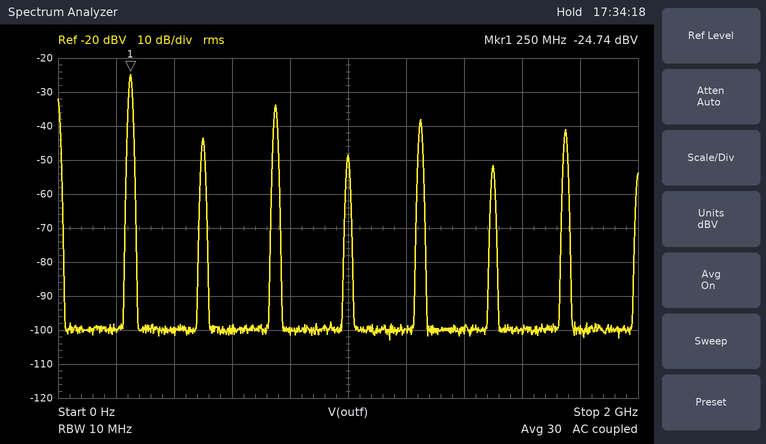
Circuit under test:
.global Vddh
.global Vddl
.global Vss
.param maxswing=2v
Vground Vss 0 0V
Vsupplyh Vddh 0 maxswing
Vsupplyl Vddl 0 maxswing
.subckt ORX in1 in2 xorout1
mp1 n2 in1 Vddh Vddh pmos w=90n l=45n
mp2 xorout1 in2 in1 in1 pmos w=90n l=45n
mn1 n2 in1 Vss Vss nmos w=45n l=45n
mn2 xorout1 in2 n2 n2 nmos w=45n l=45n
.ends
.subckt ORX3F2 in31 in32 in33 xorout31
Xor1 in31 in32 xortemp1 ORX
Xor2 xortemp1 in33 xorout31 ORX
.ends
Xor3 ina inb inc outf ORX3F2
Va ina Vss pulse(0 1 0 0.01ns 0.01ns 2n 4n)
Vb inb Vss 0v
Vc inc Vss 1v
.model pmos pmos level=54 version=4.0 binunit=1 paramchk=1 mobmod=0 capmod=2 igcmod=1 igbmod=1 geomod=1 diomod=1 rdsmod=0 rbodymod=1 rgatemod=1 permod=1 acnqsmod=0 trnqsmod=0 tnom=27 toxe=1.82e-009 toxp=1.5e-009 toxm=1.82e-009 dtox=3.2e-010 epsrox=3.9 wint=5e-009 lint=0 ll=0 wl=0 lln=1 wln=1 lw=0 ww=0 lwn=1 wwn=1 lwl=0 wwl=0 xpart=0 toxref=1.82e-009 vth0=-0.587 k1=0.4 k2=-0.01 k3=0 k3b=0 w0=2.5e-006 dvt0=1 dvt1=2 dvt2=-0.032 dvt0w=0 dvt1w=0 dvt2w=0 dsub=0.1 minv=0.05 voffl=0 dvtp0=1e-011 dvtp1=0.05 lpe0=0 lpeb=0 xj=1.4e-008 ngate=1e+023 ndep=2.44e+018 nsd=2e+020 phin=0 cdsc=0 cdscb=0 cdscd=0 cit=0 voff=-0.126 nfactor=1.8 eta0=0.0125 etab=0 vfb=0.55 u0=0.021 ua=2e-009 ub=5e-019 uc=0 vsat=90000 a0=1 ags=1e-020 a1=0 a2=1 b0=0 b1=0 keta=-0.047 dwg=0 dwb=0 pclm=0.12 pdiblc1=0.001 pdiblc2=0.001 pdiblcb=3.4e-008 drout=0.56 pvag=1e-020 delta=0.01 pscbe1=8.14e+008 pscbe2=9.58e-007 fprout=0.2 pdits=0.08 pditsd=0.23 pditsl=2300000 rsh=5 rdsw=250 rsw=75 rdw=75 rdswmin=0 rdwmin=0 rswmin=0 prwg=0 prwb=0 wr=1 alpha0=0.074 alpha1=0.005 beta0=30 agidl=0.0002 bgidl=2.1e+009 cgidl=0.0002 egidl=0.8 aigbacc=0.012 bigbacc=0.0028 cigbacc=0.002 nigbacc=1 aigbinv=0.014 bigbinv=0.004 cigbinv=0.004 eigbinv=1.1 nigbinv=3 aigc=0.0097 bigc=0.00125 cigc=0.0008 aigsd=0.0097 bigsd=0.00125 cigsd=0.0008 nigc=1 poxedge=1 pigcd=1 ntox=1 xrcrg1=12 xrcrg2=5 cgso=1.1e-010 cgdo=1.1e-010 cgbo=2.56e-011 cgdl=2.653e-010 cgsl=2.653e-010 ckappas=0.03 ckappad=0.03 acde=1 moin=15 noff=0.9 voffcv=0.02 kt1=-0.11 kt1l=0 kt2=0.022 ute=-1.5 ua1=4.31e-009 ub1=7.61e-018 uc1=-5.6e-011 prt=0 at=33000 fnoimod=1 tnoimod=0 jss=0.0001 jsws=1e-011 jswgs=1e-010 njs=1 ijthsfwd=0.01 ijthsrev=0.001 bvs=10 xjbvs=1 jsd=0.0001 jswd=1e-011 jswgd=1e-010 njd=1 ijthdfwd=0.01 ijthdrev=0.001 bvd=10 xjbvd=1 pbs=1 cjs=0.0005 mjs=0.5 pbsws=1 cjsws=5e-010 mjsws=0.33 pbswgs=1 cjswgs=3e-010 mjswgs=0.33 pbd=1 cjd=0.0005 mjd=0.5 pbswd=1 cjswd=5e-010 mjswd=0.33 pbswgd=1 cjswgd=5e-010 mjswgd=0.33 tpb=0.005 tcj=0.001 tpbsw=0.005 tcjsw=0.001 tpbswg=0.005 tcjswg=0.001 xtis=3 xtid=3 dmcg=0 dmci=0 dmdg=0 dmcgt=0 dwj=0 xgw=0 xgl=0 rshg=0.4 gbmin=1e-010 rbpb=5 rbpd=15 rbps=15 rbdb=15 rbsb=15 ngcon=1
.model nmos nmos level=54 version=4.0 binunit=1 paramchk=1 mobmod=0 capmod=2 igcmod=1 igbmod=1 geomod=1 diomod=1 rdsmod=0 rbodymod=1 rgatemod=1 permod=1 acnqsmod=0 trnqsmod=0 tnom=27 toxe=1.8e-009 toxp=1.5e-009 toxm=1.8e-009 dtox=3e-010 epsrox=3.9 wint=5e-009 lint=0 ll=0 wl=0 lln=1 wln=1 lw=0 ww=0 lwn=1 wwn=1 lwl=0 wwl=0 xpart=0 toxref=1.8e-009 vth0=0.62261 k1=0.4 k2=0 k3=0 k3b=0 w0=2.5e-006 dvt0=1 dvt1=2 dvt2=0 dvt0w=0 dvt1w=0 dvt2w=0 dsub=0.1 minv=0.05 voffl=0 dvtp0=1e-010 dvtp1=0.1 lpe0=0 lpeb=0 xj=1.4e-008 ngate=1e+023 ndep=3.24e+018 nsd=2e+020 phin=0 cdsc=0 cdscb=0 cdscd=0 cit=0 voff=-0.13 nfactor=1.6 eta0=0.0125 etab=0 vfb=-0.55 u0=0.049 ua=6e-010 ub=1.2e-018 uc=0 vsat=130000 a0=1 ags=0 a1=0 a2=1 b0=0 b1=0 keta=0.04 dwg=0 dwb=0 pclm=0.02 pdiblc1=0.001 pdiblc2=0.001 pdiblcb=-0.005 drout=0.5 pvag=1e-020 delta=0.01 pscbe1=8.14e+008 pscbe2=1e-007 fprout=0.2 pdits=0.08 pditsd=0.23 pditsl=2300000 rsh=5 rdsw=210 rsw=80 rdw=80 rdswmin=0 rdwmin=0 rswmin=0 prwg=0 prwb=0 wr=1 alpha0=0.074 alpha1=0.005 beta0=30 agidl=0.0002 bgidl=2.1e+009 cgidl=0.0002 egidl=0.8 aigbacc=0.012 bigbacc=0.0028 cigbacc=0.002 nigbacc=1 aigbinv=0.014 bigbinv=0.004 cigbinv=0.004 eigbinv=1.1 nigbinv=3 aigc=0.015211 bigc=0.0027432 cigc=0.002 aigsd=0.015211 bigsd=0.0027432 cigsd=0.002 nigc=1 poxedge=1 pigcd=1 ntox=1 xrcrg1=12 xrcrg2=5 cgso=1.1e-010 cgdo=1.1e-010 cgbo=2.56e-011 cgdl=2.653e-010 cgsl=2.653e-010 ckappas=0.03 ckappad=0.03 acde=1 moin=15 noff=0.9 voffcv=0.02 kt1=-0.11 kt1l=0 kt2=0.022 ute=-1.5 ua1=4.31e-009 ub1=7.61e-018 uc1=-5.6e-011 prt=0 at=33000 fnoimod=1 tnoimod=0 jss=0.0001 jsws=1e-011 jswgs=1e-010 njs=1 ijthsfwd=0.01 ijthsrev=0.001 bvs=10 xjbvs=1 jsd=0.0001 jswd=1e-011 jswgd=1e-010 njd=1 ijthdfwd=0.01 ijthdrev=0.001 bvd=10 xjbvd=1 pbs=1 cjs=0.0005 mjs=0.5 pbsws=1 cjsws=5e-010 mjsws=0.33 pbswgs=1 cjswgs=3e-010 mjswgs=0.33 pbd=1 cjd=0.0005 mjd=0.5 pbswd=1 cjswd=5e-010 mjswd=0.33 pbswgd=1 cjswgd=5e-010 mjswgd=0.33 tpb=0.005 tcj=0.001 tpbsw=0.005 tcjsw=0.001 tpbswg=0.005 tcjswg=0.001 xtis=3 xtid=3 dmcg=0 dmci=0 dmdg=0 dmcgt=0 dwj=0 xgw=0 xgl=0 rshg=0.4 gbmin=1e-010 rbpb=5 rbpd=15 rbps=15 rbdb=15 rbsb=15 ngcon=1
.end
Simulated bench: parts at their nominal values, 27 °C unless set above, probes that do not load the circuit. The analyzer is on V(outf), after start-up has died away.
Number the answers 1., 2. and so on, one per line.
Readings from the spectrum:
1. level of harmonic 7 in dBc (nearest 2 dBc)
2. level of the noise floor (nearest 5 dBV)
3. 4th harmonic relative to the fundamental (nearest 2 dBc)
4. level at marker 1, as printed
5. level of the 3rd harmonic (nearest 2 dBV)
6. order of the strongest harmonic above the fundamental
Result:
1. -16 dBc
2. -100 dBV
3. -24 dBc
4. -24.74 dBV
5. -34 dBV
6. 3
